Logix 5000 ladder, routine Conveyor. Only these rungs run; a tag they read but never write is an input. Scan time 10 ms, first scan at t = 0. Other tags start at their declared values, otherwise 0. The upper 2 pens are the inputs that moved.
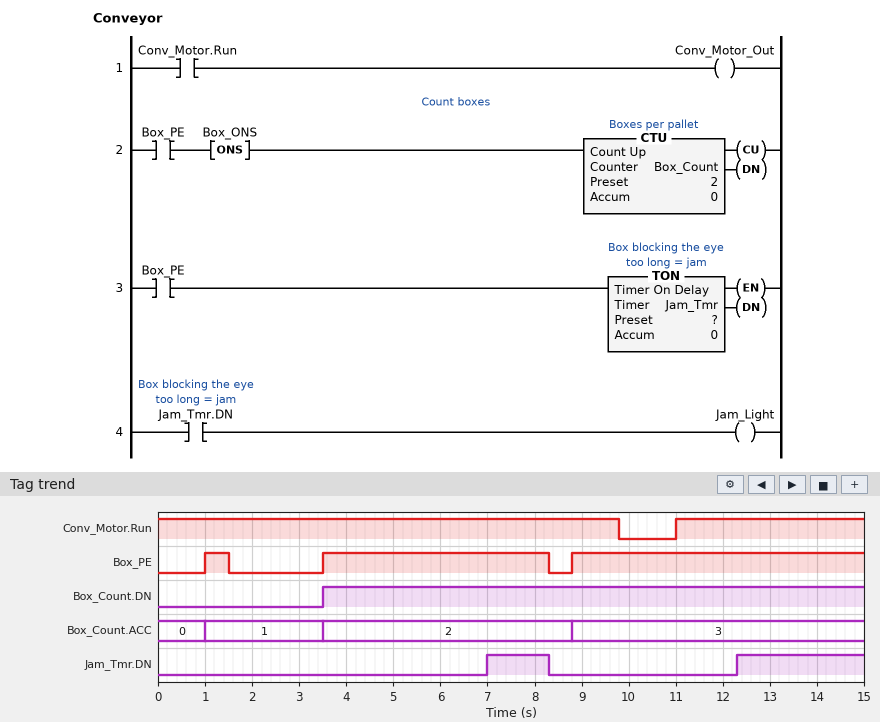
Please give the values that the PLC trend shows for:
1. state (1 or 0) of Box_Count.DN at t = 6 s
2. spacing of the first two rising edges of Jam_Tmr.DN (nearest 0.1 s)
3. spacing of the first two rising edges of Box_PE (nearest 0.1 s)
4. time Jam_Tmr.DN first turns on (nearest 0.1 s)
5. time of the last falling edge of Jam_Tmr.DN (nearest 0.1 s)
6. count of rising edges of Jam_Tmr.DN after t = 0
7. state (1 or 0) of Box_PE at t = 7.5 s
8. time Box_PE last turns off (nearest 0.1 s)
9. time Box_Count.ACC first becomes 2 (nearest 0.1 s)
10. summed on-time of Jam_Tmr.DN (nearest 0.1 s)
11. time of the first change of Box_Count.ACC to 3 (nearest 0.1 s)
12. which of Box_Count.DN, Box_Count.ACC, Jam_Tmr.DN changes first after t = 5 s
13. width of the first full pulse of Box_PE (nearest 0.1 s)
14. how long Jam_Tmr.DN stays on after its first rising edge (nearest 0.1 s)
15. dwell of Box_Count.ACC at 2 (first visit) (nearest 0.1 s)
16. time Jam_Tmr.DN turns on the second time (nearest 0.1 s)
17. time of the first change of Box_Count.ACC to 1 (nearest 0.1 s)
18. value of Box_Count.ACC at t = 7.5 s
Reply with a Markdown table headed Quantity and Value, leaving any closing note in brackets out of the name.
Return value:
| Quantity | Value |
|---|---|
| state (1 or 0) of Box_Count.DN at t = 6 s | 1 |
| spacing of the first two rising edges of Jam_Tmr.DN | 5.3 s |
| spacing of the first two rising edges of Box_PE | 2.5 s |
| time Jam_Tmr.DN first turns on | 7.0 s |
| time of the last falling edge of Jam_Tmr.DN | 8.3 s |
| count of rising edges of Jam_Tmr.DN after t = 0 | 2 |
| state (1 or 0) of Box_PE at t = 7.5 s | 1 |
| time Box_PE last turns off | 8.3 s |
| time Box_Count.ACC first becomes 2 | 3.5 s |
| summed on-time of Jam_Tmr.DN | 4.0 s |
| time of the first change of Box_Count.ACC to 3 | 8.8 s |
| which of Box_Count.DN, Box_Count.ACC, Jam_Tmr.DN changes first after t = 5 s | Jam_Tmr.DN |
| width of the first full pulse of Box_PE | 0.5 s |
| how long Jam_Tmr.DN stays on after its first rising edge | 1.3 s |
| dwell of Box_Count.ACC at 2 (first visit) | 5.3 s |
| time Jam_Tmr.DN turns on the second time | 12.3 s |
| time of the first change of Box_Count.ACC to 1 | 1.0 s |
| value of Box_Count.ACC at t = 7.5 s | 2 |
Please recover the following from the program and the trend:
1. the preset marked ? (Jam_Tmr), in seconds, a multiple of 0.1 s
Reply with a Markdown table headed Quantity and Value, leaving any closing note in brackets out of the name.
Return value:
| Quantity | Value |
|---|---|
| the preset marked ? (Jam_Tmr), in seconds, a multiple of 0.1 s | 3.5 s |
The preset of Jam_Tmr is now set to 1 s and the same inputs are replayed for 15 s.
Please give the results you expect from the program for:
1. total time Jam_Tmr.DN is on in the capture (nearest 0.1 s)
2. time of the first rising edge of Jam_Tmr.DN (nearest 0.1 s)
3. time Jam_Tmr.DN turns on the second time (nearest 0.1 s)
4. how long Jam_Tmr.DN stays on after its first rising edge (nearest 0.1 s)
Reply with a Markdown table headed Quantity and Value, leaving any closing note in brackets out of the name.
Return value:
| Quantity | Value |
|---|---|
| total time Jam_Tmr.DN is on in the capture | 9.0 s |
| time of the first rising edge of Jam_Tmr.DN | 4.5 s |
| time Jam_Tmr.DN turns on the second time | 9.8 s |
| how long Jam_Tmr.DN stays on after its first rising edge | 3.8 s |
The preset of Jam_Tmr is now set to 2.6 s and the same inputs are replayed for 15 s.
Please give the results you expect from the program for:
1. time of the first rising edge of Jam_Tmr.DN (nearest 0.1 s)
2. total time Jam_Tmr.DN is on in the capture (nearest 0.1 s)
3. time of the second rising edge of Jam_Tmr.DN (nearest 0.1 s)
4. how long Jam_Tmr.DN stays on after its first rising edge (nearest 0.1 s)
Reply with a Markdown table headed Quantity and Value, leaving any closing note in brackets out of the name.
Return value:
| Quantity | Value |
|---|---|
| time of the first rising edge of Jam_Tmr.DN | 6.1 s |
| total time Jam_Tmr.DN is on in the capture | 5.8 s |
| time of the second rising edge of Jam_Tmr.DN | 11.4 s |
| how long Jam_Tmr.DN stays on after its first rising edge | 2.2 s |
